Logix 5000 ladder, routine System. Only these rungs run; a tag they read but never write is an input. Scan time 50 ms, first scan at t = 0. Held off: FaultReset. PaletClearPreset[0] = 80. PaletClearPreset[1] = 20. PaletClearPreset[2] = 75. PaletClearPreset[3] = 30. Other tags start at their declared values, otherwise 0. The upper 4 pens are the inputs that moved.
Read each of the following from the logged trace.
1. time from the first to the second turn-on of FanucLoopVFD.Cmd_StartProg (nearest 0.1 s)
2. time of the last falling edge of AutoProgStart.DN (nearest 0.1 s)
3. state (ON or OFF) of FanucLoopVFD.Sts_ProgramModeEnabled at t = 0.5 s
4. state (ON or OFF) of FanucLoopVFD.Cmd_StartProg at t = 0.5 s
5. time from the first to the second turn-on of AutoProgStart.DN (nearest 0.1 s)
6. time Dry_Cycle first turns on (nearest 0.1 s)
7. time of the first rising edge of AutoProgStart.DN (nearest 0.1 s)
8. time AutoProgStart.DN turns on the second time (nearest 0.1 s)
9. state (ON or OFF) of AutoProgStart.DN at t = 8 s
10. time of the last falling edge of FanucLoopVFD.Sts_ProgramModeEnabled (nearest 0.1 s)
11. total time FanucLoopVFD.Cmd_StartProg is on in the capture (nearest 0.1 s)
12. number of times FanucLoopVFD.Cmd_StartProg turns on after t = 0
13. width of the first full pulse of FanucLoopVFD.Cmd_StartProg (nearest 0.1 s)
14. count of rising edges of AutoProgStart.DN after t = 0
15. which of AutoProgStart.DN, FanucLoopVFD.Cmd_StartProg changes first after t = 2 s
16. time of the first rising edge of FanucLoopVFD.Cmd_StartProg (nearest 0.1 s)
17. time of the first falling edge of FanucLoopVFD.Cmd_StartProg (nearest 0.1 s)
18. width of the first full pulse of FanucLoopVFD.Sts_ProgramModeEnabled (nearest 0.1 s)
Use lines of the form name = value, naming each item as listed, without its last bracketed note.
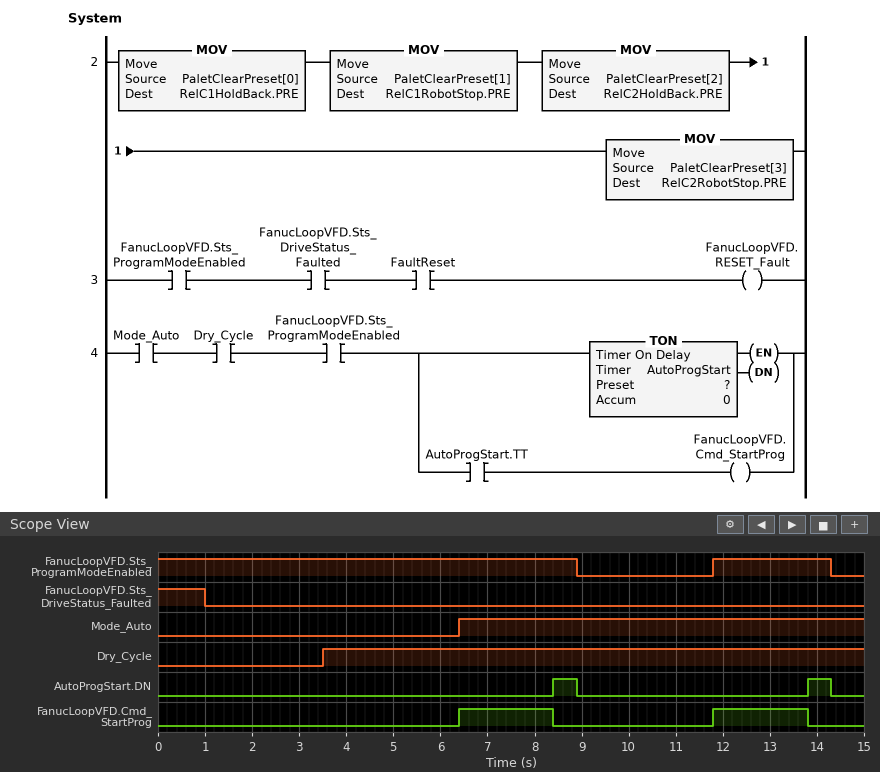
time from the first to the second turn-on of FanucLoopVFD.Cmd_StartProg = 5.4 s
time of the last falling edge of AutoProgStart.DN = 14.3 s
state (ON or OFF) of FanucLoopVFD.Sts_ProgramModeEnabled at t = 0.5 s = ON
state (ON or OFF) of FanucLoopVFD.Cmd_StartProg at t = 0.5 s = OFF
time from the first to the second turn-on of AutoProgStart.DN = 5.4 s
time Dry_Cycle first turns on = 3.5 s
time of the first rising edge of AutoProgStart.DN = 8.4 s
time AutoProgStart.DN turns on the second time = 13.8 s
state (ON or OFF) of AutoProgStart.DN at t = 8 s = OFF
time of the last falling edge of FanucLoopVFD.Sts_ProgramModeEnabled = 14.3 s
total time FanucLoopVFD.Cmd_StartProg is on in the capture = 4.0 s
number of times FanucLoopVFD.Cmd_StartProg turns on after t = 0 = 2
width of the first full pulse of FanucLoopVFD.Cmd_StartProg = 2.0 s
count of rising edges of AutoProgStart.DN after t = 0 = 2
which of AutoProgStart.DN, FanucLoopVFD.Cmd_StartProg changes first after t = 2 s = FanucLoopVFD.Cmd_StartProg
time of the first rising edge of FanucLoopVFD.Cmd_StartProg = 6.4 s
time of the first falling edge of FanucLoopVFD.Cmd_StartProg = 8.4 s
width of the first full pulse of FanucLoopVFD.Sts_ProgramModeEnabled = 2.5 s
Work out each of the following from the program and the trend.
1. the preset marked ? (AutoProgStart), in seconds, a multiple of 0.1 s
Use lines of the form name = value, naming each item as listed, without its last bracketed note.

the preset marked ? (AutoProgStart), in seconds, a multiple of 0.1 s = 2.0 s
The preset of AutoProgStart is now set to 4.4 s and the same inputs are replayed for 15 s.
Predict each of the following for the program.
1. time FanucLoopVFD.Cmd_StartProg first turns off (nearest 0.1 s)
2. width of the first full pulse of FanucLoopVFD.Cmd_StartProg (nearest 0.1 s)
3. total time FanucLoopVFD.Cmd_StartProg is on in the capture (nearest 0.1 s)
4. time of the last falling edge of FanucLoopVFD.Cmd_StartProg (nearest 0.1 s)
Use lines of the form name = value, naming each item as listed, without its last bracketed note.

time FanucLoopVFD.Cmd_StartProg first turns off = 8.9 s
width of the first full pulse of FanucLoopVFD.Cmd_StartProg = 2.5 s
total time FanucLoopVFD.Cmd_StartProg is on in the capture = 5.0 s
time of the last falling edge of FanucLoopVFD.Cmd_StartProg = 14.3 s
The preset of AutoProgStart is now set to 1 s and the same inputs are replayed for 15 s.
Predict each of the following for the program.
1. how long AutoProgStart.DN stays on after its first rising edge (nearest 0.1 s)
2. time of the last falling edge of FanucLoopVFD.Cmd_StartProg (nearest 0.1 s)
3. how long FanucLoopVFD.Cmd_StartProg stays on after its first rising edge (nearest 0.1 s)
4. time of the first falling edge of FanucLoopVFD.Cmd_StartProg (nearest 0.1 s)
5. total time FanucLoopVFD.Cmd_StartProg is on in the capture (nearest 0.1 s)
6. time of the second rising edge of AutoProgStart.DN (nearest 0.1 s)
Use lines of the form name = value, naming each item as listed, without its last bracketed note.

how long AutoProgStart.DN stays on after its first rising edge = 1.5 s
time of the last falling edge of FanucLoopVFD.Cmd_StartProg = 12.8 s
how long FanucLoopVFD.Cmd_StartProg stays on after its first rising edge = 1.0 s
time of the first falling edge of FanucLoopVFD.Cmd_StartProg = 7.4 s
total time FanucLoopVFD.Cmd_StartProg is on in the capture = 2.0 s
time of the second rising edge of AutoProgStart.DN = 12.8 s
